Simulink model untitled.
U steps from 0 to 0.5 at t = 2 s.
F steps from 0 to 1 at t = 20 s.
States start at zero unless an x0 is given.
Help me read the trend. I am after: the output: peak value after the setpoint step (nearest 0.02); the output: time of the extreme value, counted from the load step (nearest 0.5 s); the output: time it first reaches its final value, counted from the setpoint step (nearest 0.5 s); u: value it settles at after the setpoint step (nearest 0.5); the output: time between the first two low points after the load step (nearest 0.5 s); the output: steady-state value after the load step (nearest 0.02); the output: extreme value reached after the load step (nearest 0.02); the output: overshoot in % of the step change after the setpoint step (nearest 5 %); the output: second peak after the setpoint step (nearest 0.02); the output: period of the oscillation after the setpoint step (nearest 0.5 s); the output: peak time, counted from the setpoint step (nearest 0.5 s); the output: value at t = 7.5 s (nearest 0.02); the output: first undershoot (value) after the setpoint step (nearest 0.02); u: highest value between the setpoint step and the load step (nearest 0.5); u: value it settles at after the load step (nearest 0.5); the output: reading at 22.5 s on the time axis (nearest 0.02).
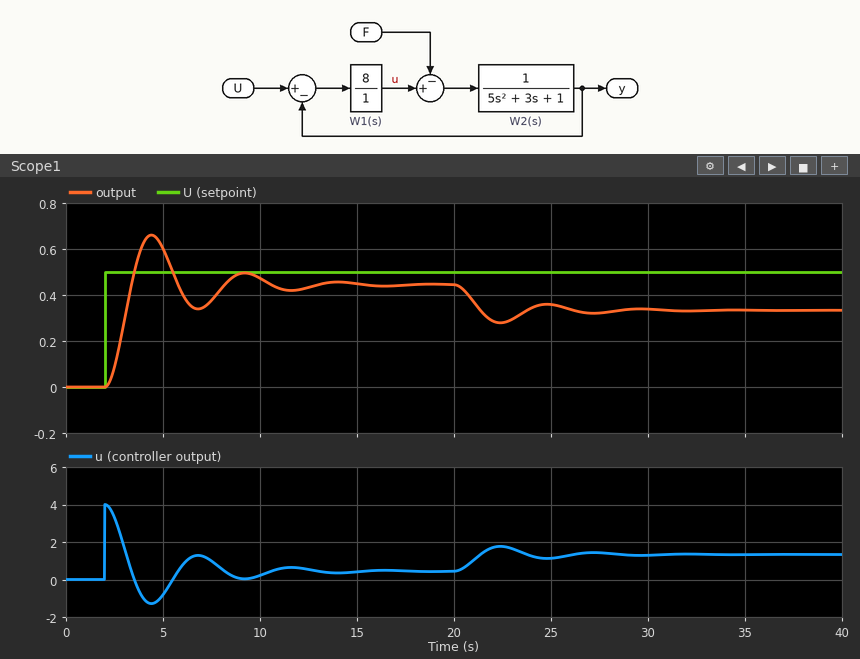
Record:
0.66
2.5 s
1.5 s
0.5
5.0 s
0.34
0.28
50 %
0.50
5.0 s
2.5 s
0.38
0.34
4.0
1.5
0.28
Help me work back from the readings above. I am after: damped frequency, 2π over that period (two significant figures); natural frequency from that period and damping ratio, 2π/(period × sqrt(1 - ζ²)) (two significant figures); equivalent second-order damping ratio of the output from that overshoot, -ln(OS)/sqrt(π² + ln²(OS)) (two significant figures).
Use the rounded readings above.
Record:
1.3 rad/s
1.3 rad/s
0.22
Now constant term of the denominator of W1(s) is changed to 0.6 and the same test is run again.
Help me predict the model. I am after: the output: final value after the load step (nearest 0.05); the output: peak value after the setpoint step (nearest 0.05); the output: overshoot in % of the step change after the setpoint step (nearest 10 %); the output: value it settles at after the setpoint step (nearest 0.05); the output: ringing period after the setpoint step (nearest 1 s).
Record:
0.40
0.75
60 %
0.45
4 s
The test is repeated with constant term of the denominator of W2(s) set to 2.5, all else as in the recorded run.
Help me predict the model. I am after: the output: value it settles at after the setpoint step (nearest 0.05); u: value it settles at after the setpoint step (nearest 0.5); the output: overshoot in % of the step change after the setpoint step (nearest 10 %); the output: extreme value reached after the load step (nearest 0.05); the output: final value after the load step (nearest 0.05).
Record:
0.40
1.0
50 %
0.25
0.30
